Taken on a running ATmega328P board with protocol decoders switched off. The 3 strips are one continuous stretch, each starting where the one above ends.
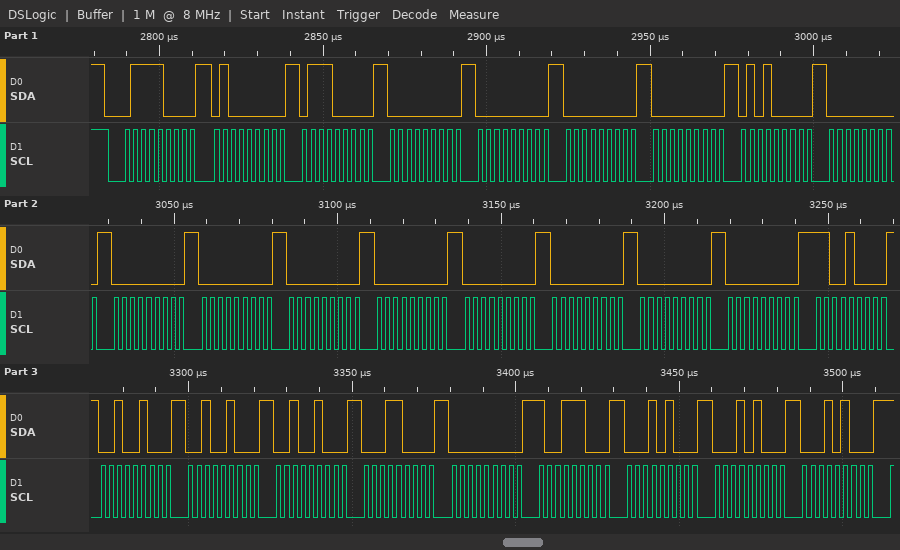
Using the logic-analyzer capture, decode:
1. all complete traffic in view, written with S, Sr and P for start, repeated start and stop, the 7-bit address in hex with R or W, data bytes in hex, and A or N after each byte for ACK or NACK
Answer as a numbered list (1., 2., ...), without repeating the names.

1. S 3CW A 40 A 70 A 00 A 00 A 00 A 00 A 50 A 00 A 00 A 00 A 00 A 00 A 00 A 00 A 00 A 00 A C8 A 24 A 24 A 24 A 18 A 00 A 9C A 14 A 14 A 14 A
